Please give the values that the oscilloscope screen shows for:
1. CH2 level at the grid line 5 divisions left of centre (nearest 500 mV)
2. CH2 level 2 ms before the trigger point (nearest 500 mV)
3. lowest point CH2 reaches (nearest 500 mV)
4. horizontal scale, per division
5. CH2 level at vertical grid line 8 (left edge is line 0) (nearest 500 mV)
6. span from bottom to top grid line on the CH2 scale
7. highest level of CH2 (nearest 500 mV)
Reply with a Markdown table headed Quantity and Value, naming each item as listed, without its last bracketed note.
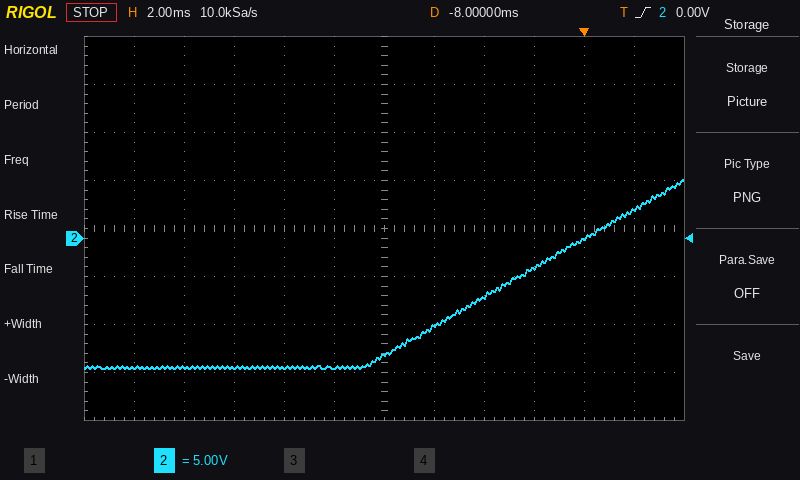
| Quantity | Value |
|---|---|
| CH2 level at the grid line 5 divisions left of centre | -13.5 V |
| CH2 level 2 ms before the trigger point | -3.0 V |
| lowest point CH2 reaches | -13.5 V |
| horizontal scale, per division | 2 ms |
| CH2 level at vertical grid line 8 (left edge is line 0) | -6.0 V |
| span from bottom to top grid line on the CH2 scale | 40 V |
| highest level of CH2 | 6.0 V |
